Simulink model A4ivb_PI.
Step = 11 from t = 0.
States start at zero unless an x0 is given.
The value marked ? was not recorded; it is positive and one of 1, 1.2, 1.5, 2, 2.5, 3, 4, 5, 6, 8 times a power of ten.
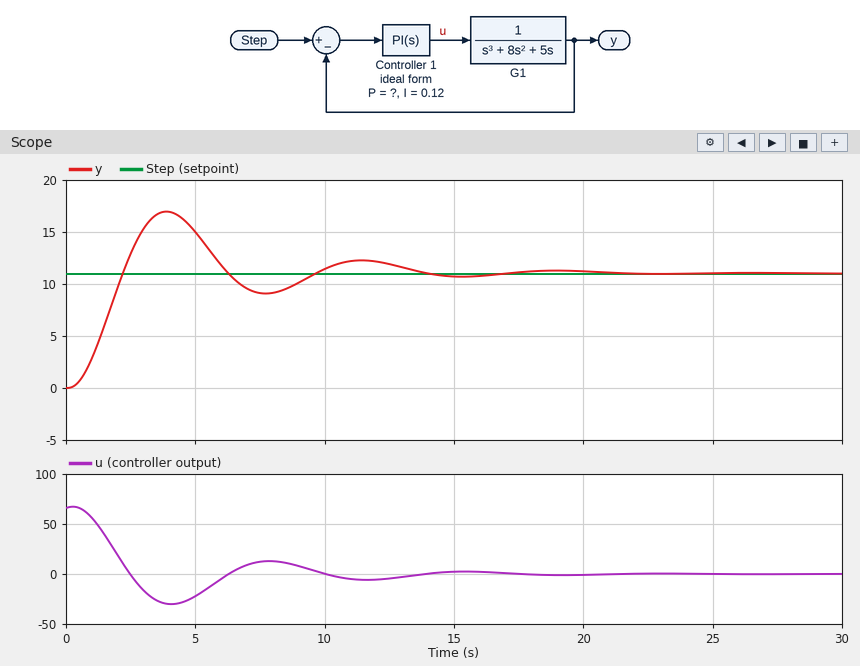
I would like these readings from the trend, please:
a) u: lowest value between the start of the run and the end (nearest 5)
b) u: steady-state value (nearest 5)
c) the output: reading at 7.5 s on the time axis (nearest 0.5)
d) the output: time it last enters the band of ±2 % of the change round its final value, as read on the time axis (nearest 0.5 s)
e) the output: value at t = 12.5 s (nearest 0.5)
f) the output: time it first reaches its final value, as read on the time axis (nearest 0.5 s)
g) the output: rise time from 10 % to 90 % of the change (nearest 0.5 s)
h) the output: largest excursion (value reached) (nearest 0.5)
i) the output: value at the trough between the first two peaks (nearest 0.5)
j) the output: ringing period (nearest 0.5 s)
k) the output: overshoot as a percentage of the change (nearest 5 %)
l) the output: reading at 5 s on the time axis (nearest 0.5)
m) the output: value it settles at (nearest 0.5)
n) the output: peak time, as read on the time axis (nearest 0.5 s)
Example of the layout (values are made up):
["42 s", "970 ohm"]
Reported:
["-30", "0", "9.0", "20.0 s", "12.0", "2.0 s", "1.5 s", "17.0", "9.0", "7.5 s", "55 %", "15.0", "11.0", "4.0 s"]
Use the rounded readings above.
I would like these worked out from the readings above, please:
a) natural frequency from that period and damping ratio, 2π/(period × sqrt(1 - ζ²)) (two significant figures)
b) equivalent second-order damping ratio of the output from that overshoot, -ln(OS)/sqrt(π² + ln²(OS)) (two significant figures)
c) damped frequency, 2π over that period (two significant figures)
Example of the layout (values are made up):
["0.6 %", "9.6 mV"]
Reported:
["0.85 rad/s", "0.19", "0.84 rad/s"]
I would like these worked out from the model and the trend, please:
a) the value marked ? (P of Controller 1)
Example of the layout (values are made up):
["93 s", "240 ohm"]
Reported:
["6"]
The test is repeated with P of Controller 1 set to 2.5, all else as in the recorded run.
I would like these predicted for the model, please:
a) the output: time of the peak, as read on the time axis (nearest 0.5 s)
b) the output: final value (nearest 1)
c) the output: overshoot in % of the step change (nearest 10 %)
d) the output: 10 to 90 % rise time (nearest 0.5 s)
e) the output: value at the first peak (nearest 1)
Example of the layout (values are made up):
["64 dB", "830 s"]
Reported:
["6.5 s", "11", "40 %", "2.5 s", "15"]
